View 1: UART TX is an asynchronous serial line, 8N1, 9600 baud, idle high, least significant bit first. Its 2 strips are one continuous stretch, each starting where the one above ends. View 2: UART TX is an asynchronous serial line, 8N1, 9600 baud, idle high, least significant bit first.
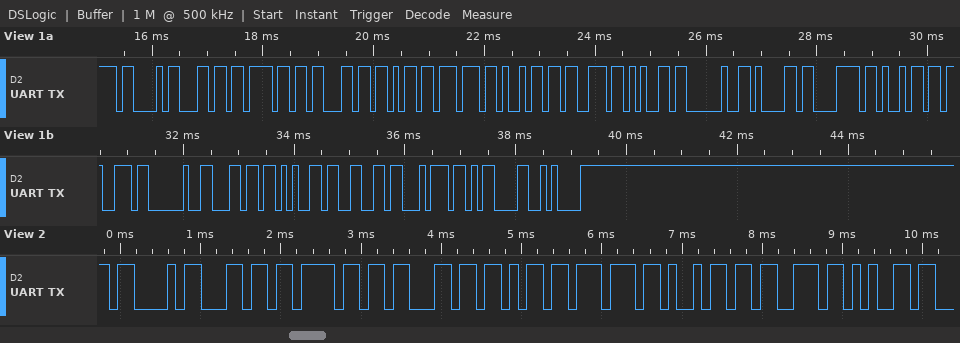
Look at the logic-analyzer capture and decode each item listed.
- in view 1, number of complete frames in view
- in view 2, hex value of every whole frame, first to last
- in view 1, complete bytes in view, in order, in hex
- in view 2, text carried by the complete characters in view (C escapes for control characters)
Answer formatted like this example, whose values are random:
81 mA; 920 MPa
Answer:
21; 43 6C 6F 63 6B 77 69 73 65; 43 6C 6F 63 6B 77 69 73 65 20 61 78 69 73 20 6C 65 66 74 0D 0A; "Clockwise"
